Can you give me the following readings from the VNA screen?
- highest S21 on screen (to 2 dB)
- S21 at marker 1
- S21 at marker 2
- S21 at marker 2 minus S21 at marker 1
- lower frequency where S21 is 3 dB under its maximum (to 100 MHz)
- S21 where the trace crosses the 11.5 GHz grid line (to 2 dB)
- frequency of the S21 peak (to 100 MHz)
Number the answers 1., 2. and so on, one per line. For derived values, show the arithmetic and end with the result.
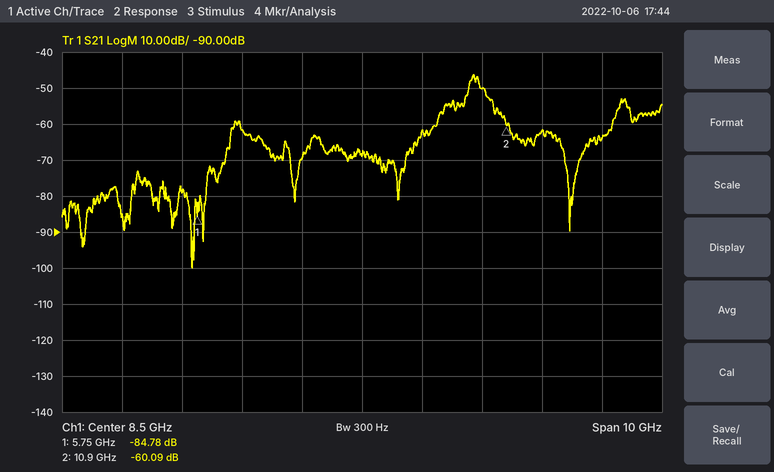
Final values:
1. -46 dB
2. -84.78 dB
3. -60.09 dB
4. -60.09 − (-84.78) = 24.69 dB
5. 10.3 GHz
6. -62 dB
7. 10.4 GHz
